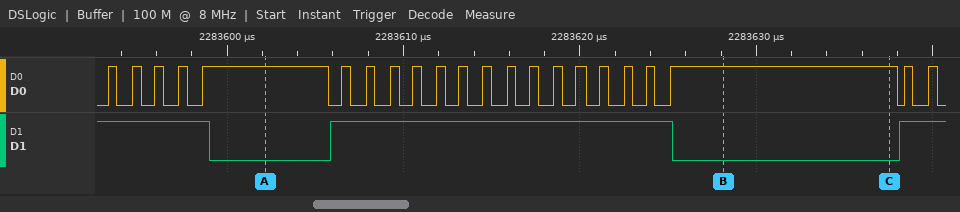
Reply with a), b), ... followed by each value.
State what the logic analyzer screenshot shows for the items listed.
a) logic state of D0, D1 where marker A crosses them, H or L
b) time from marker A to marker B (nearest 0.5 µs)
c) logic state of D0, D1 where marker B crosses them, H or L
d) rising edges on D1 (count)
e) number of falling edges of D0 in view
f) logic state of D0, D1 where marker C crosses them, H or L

a) D0=H, D1=L
b) 26 µs
c) D0=H, D1=L
d) 2
e) 22
f) D0=H, D1=L
